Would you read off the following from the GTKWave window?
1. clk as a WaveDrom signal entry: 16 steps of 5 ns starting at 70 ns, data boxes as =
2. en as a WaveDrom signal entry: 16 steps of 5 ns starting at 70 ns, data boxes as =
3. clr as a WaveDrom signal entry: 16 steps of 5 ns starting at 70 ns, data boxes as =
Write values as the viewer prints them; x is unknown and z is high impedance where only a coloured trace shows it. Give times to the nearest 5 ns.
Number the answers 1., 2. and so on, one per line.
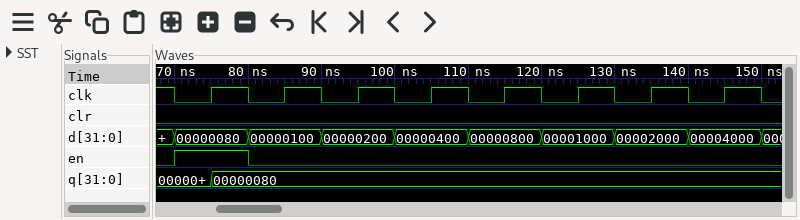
1. {name: 'clk', wave: '0101010101010101'}
2. {name: 'en', wave: '1.0.............'}
3. {name: 'clr', wave: '0...............'}
